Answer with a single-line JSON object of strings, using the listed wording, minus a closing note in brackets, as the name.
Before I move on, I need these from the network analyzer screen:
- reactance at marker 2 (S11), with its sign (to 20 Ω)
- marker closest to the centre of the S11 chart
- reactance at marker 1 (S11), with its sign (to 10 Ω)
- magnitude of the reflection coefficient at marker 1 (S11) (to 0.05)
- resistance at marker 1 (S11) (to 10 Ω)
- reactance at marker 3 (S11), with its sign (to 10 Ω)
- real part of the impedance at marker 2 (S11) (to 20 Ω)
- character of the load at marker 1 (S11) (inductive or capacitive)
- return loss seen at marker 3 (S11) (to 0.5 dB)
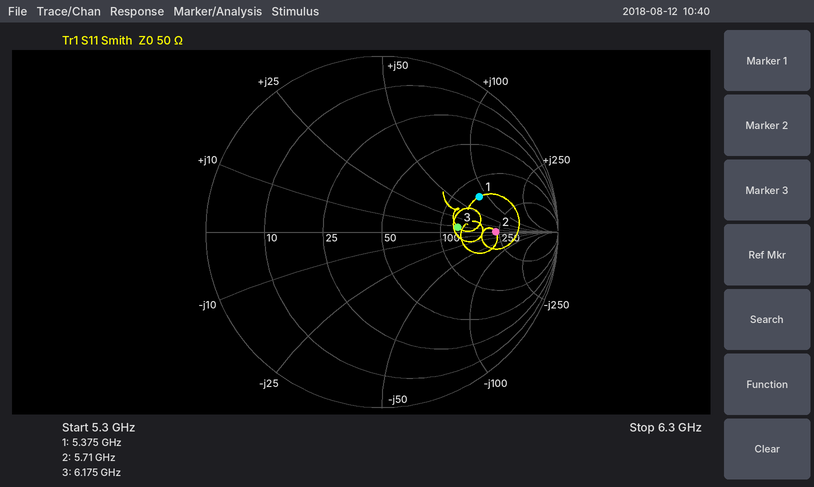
{"reactance at marker 2 (S11), with its sign": "0 Ω", "marker closest to the centre of the S11 chart": "marker 3", "reactance at marker 1 (S11), with its sign": "+80 Ω", "magnitude of the reflection coefficient at marker 1 (S11)": "0.60", "resistance at marker 1 (S11)": "140 Ω", "reactance at marker 3 (S11), with its sign": "+10 Ω", "real part of the impedance at marker 2 (S11)": "240 Ω", "character of the load at marker 1 (S11)": "inductive", "return loss seen at marker 3 (S11)": "7.5 dB"}
